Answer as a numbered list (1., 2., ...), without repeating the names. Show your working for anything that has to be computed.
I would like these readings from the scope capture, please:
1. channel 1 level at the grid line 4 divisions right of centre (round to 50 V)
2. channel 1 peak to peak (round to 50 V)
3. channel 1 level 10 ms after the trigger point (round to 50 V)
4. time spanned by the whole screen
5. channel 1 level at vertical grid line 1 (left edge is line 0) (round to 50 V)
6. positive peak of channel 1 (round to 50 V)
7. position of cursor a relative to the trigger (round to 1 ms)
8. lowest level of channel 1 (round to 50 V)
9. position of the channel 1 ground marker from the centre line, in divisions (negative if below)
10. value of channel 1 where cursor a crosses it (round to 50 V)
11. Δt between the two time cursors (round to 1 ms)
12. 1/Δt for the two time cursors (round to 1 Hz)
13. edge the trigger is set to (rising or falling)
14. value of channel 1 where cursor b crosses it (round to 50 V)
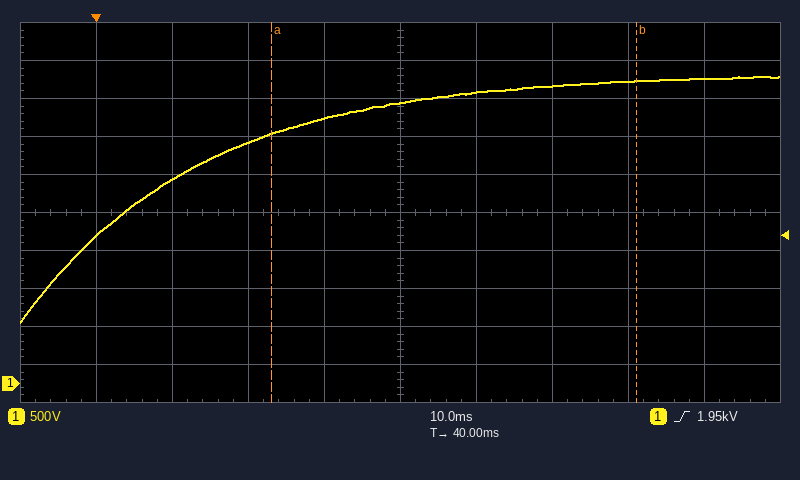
1. 4.00 kV
2. 4.05 kV − (800 V) = 3.25 kV
3. 2.70 kV
4. 100 ms
5. 1.95 kV
6. 4.05 kV
7. +23 ms
8. 800 V
9. -4.5 div
10. 3.30 kV
11. 48 ms
12. 1 / 48 ms ≈ 21 Hz
13. rising
14. 4.00 kV
